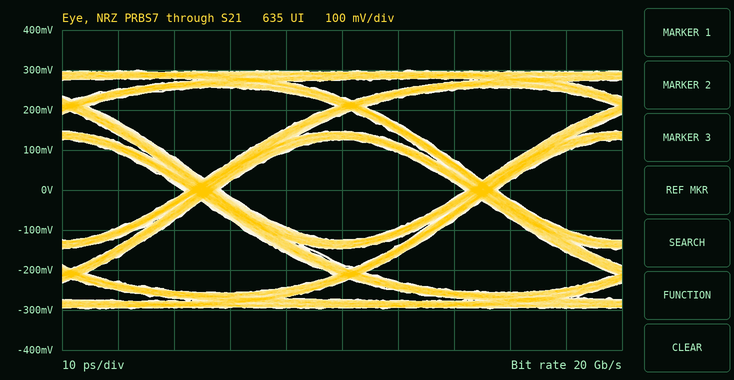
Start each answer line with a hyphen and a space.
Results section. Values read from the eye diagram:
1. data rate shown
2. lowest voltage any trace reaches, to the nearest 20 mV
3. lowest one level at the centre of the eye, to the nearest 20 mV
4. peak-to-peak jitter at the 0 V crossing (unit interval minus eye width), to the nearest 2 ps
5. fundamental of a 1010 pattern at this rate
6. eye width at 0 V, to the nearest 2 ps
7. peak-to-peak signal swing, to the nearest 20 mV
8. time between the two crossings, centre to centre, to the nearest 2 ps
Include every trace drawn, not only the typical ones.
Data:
- 20 Gb/s
- -300 mV
- 120 mV
- 6 ps
- 10 GHz
- 44 ps
- 600 mV
- 50 ps
